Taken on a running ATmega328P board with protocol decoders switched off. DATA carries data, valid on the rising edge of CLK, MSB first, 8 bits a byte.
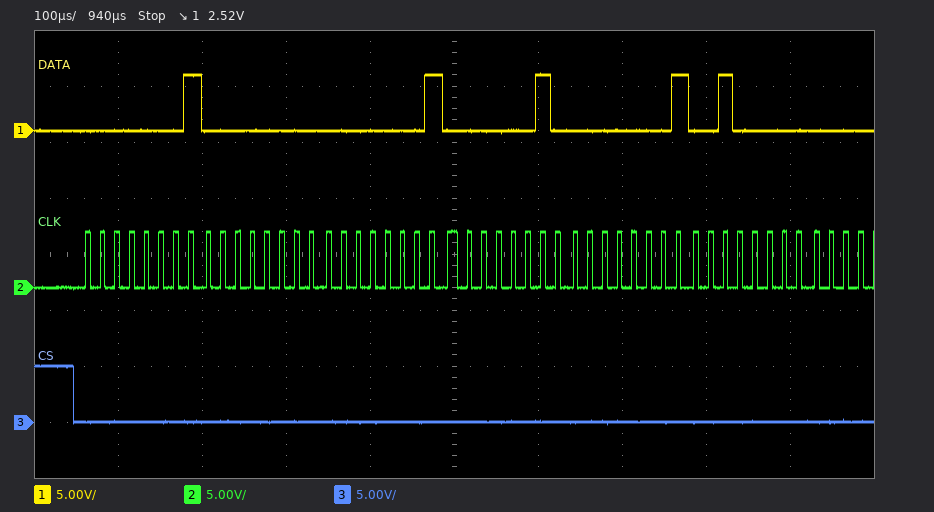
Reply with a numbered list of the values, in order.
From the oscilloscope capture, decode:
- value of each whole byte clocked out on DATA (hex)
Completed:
1. 0x01 0x00 0x01 0x02 0x01 0x20
